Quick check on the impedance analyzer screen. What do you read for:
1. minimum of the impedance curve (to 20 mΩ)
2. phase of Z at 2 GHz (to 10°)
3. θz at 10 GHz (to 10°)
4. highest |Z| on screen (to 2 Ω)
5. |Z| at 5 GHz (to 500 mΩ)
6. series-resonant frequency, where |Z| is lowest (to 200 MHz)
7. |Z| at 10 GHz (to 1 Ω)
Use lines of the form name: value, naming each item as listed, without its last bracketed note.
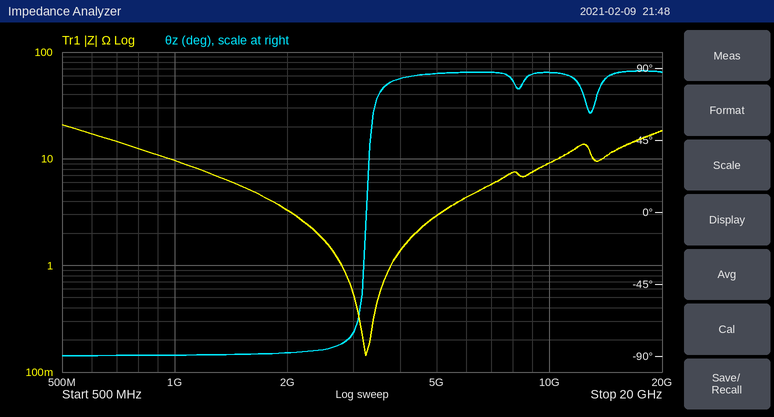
minimum of the impedance curve: 140 mΩ
phase of Z at 2 GHz: -90°
θz at 10 GHz: 90°
highest |Z| on screen: 20 Ω
|Z| at 5 GHz: 3.0 Ω
series-resonant frequency, where |Z| is lowest: 3.2 GHz
|Z| at 10 GHz: 9 Ω
